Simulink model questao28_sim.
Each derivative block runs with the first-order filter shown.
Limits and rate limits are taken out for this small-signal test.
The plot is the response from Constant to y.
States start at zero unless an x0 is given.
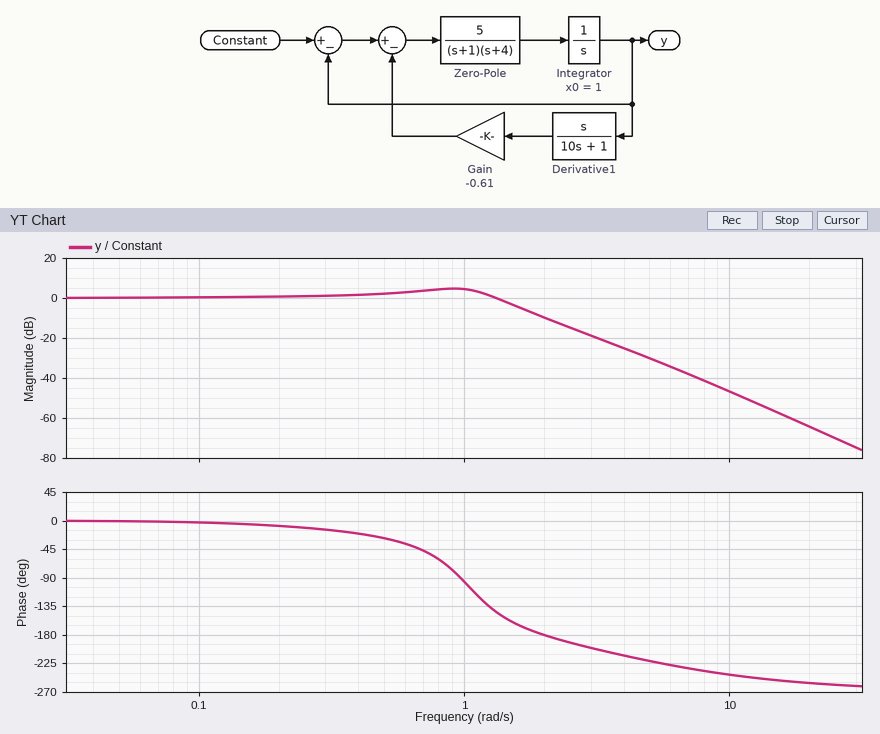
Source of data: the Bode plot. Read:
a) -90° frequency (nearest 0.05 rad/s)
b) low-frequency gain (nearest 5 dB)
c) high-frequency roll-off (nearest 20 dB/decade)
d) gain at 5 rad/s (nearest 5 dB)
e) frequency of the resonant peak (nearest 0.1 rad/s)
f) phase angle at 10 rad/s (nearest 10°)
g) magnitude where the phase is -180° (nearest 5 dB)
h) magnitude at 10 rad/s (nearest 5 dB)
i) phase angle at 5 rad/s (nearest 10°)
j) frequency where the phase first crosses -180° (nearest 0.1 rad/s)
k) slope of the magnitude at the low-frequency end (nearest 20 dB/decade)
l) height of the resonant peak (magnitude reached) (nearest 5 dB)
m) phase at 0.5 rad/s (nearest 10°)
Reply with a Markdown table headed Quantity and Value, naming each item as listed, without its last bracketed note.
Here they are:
| Quantity | Value |
|---|---|
| -90° frequency | 0.95 rad/s |
| low-frequency gain | 0 dB |
| high-frequency roll-off | -60 dB/decade |
| gain at 5 rad/s | -30 dB |
| frequency of the resonant peak | 0.9 rad/s |
| phase angle at 10 rad/s | -240° |
| magnitude where the phase is -180° | -10 dB |
| magnitude at 10 rad/s | -45 dB |
| phase angle at 5 rad/s | -220° |
| frequency where the phase first crosses -180° | 2.0 rad/s |
| slope of the magnitude at the low-frequency end | 0 dB/decade |
| height of the resonant peak (magnitude reached) | 5 dB |
| phase at 0.5 rad/s | -30° |
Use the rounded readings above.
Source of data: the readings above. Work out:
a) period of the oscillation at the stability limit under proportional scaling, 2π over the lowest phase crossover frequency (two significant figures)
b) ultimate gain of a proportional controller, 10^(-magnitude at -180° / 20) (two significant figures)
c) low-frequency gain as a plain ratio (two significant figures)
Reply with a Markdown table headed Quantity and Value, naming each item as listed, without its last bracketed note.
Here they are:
| Quantity | Value |
|---|---|
| period of the oscillation at the stability limit under proportional scaling, 2π over the lowest phase crossover frequency | 3.1 s |
| ultimate gain of a proportional controller, 10^(-magnitude at -180° / 20) | 3.2 |
| low-frequency gain as a plain ratio | 1.0 |
